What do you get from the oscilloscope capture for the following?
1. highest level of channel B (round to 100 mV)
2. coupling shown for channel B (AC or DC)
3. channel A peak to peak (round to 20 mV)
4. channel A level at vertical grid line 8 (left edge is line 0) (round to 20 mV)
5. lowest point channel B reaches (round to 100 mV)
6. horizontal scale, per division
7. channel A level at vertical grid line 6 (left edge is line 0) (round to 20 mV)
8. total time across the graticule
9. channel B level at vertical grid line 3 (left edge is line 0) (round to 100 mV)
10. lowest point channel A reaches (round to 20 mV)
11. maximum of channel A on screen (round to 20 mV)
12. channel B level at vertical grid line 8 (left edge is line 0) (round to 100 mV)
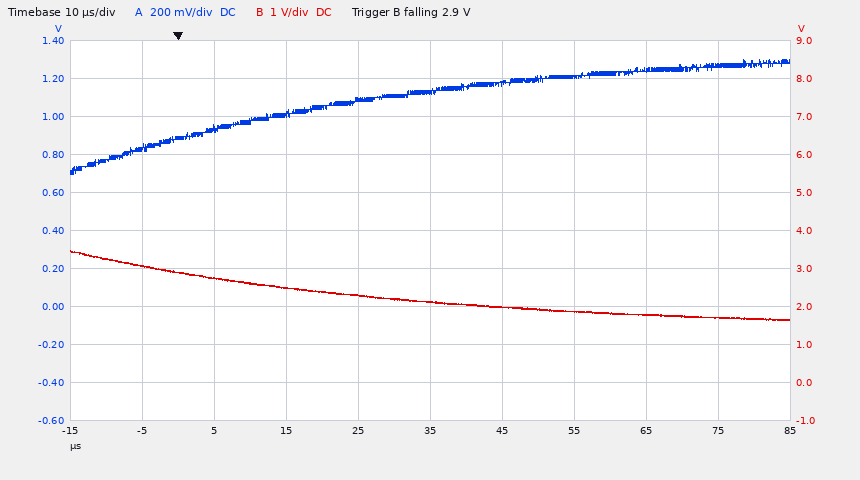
3.5 V
DC
600 mV
1.24 V
1.6 V
10 µs
1.18 V
100 µs
2.5 V
700 mV
1.30 V
1.8 V
